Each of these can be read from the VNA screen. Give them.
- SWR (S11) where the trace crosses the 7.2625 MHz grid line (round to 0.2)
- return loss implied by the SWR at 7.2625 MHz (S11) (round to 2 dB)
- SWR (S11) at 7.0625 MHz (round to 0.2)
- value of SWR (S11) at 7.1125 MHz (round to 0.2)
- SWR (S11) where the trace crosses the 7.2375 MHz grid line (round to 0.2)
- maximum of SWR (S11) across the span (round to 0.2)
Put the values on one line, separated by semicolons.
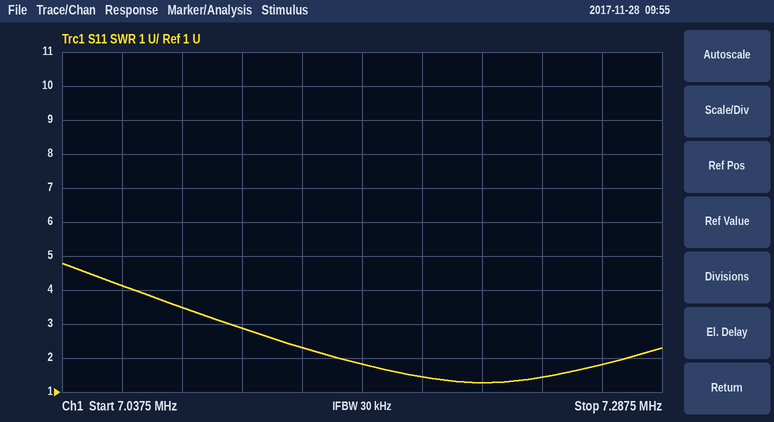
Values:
1.8; 10 dB; 4.2; 2.8; 1.4; 4.8
